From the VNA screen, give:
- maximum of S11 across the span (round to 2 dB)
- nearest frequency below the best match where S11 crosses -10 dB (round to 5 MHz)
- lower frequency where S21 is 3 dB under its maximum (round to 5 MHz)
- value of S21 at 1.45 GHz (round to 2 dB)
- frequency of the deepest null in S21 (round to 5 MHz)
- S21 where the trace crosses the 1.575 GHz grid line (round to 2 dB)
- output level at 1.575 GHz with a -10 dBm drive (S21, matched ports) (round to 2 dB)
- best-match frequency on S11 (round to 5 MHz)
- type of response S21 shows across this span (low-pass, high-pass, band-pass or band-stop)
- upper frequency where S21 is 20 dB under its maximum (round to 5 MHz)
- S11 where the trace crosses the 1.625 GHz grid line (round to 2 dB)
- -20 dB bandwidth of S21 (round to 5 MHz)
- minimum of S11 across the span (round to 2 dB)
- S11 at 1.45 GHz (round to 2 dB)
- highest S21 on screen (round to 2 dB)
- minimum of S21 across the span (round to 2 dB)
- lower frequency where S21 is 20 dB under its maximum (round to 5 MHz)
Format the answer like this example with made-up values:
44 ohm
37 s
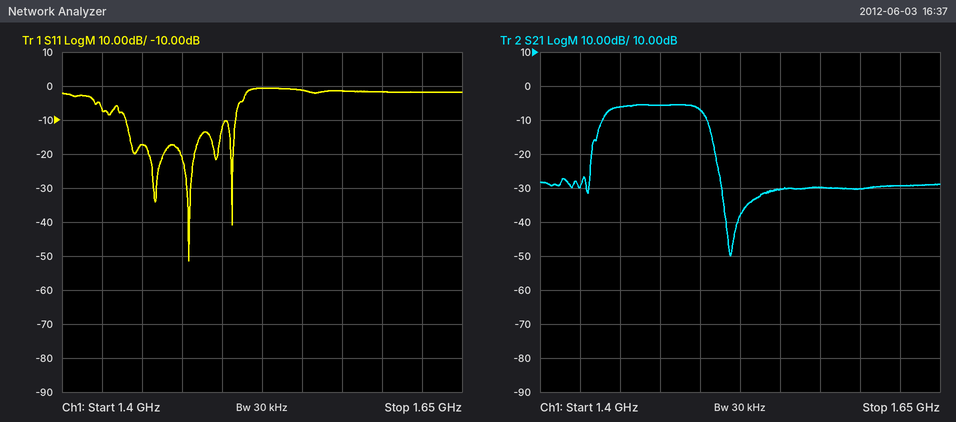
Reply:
0 dB
1.440 GHz
1.440 GHz
-6 dB
1.520 GHz
-30 dB
-40 dBm
1.480 GHz
band-pass
1.510 GHz
-2 dB
80 MHz
-52 dB
-18 dB
-6 dB
-50 dB
1.430 GHz
